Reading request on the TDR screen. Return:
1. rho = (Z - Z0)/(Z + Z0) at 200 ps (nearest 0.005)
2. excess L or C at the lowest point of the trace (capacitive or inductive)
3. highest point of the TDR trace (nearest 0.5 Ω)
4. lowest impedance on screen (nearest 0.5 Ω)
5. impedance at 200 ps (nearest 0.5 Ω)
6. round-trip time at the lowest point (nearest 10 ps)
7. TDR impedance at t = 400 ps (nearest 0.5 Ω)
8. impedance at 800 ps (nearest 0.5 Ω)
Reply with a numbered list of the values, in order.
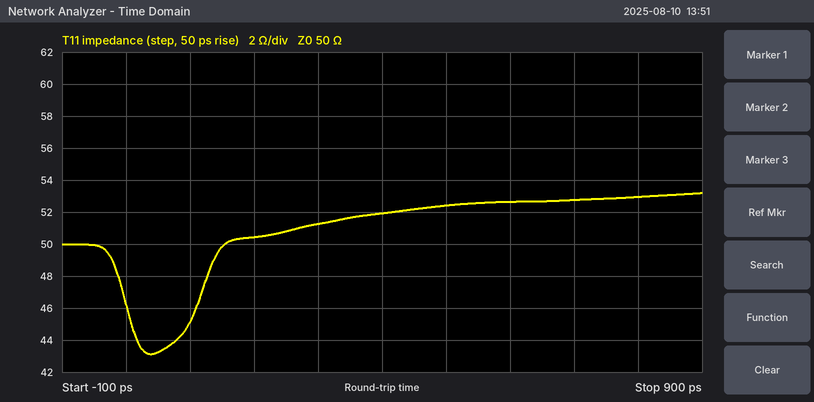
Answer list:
1. +0.005
2. capacitive
3. 53.0 Ω
4. 43.0 Ω
5. 50.5 Ω
6. 40 ps
7. 52.0 Ω
8. 53.0 Ω
